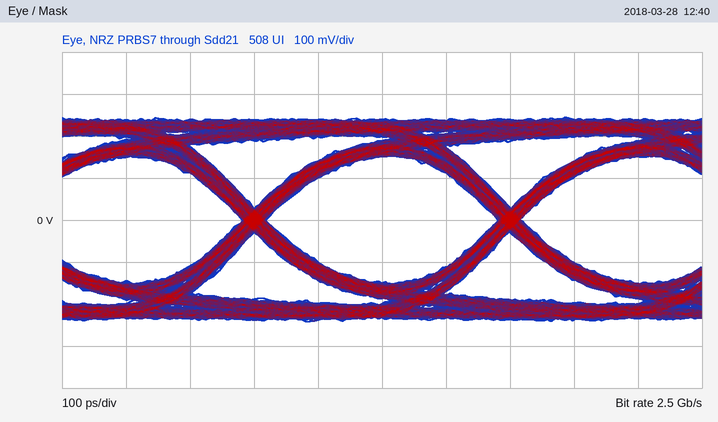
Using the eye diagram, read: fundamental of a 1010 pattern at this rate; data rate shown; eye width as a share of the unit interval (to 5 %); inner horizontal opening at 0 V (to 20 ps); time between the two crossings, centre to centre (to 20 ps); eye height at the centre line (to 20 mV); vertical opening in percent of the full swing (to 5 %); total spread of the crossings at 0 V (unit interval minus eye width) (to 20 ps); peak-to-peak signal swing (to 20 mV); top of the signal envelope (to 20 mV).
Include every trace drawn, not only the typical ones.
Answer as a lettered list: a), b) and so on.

a) 1.25 GHz
b) 2.5 Gb/s
c) 90 %
d) 360 ps
e) 400 ps
f) 300 mV
g) 60 %
h) 40 ps
i) 480 mV
j) 240 mV
